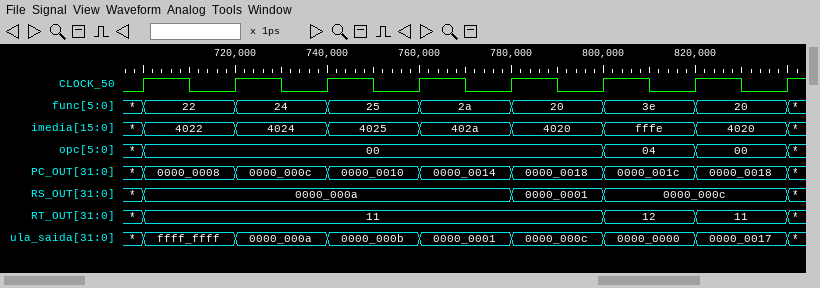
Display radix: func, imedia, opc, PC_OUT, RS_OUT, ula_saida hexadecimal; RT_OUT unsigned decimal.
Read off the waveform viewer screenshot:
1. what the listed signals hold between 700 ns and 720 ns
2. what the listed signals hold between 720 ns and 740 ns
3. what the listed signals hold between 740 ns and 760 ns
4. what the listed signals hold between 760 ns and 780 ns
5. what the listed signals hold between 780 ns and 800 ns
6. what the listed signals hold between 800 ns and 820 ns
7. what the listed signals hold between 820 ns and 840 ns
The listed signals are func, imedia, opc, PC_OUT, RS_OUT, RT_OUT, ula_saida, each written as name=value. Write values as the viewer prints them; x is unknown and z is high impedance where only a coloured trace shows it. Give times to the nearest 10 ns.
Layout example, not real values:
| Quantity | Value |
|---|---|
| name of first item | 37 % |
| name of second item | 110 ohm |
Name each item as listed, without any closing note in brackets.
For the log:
| Quantity | Value |
|---|---|
| what the listed signals hold between 700 ns and 720 ns | func=22, imedia=4022, opc=00, PC_OUT=0000_0008, RS_OUT=0000_000a, RT_OUT=11, ula_saida=ffff_ffff |
| what the listed signals hold between 720 ns and 740 ns | func=24, imedia=4024, opc=00, PC_OUT=0000_000c, RS_OUT=0000_000a, RT_OUT=11, ula_saida=0000_000a |
| what the listed signals hold between 740 ns and 760 ns | func=25, imedia=4025, opc=00, PC_OUT=0000_0010, RS_OUT=0000_000a, RT_OUT=11, ula_saida=0000_000b |
| what the listed signals hold between 760 ns and 780 ns | func=2a, imedia=402a, opc=00, PC_OUT=0000_0014, RS_OUT=0000_000a, RT_OUT=11, ula_saida=0000_0001 |
| what the listed signals hold between 780 ns and 800 ns | func=20, imedia=4020, opc=00, PC_OUT=0000_0018, RS_OUT=0000_0001, RT_OUT=11, ula_saida=0000_000c |
| what the listed signals hold between 800 ns and 820 ns | func=3e, imedia=fffe, opc=04, PC_OUT=0000_001c, RS_OUT=0000_000c, RT_OUT=12, ula_saida=0000_0000 |
| what the listed signals hold between 820 ns and 840 ns | func=20, imedia=4020, opc=00, PC_OUT=0000_0018, RS_OUT=0000_000c, RT_OUT=11, ula_saida=0000_0017 |
